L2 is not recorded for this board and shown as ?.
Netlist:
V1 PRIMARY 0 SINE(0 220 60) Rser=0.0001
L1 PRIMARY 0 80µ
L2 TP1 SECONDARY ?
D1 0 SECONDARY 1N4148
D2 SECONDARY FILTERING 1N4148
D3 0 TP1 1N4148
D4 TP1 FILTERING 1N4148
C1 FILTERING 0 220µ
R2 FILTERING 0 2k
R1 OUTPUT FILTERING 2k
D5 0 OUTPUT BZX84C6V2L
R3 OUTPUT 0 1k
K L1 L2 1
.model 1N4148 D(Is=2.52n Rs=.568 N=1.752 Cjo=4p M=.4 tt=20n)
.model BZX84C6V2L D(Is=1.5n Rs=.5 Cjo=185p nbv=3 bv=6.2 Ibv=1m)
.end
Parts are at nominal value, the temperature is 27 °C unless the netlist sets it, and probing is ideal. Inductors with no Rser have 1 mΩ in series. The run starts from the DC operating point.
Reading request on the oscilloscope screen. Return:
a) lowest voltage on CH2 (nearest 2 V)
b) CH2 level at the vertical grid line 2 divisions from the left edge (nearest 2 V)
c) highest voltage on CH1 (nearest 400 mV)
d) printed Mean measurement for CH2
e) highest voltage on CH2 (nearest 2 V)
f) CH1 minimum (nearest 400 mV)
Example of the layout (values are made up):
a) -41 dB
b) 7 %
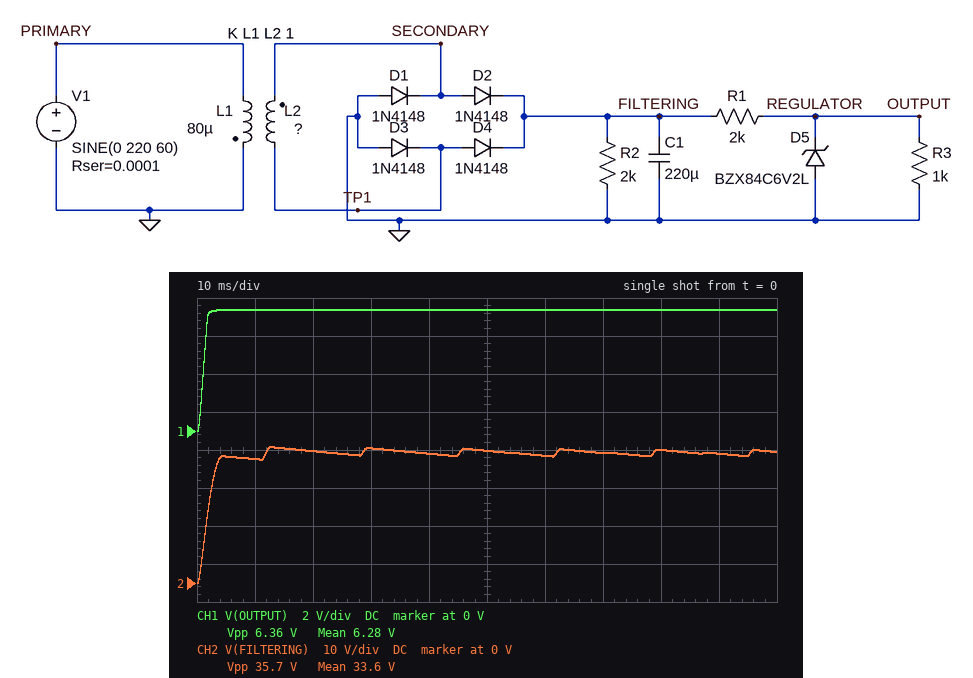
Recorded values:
a) 0 V
b) 34 V
c) 6.4 V
d) 33.6 V
e) 36 V
f) 0 V
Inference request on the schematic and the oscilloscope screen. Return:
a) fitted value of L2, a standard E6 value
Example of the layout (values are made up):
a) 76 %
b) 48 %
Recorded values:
a) 2.2 µH
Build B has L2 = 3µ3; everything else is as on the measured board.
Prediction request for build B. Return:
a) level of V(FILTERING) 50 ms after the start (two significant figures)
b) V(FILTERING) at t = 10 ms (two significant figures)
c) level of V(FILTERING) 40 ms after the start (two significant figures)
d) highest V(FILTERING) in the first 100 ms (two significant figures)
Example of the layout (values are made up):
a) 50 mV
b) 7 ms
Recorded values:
a) 43 V
b) 40 V
c) 42 V
d) 44 V
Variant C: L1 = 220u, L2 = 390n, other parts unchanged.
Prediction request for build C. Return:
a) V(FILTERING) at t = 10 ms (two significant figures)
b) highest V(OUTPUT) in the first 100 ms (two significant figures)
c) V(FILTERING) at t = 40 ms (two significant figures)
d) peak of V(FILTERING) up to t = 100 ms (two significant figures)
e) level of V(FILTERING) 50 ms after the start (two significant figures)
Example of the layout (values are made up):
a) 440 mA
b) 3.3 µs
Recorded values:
a) 7.4 V
b) 2.6 V
c) 7.6 V
d) 7.8 V
e) 7.7 V
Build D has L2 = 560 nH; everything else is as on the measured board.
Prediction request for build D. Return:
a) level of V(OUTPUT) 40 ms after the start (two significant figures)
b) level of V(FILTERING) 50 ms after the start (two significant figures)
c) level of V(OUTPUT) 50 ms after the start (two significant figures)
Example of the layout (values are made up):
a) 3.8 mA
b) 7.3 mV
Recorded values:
a) 5.5 V
b) 17 V
c) 5.6 V
